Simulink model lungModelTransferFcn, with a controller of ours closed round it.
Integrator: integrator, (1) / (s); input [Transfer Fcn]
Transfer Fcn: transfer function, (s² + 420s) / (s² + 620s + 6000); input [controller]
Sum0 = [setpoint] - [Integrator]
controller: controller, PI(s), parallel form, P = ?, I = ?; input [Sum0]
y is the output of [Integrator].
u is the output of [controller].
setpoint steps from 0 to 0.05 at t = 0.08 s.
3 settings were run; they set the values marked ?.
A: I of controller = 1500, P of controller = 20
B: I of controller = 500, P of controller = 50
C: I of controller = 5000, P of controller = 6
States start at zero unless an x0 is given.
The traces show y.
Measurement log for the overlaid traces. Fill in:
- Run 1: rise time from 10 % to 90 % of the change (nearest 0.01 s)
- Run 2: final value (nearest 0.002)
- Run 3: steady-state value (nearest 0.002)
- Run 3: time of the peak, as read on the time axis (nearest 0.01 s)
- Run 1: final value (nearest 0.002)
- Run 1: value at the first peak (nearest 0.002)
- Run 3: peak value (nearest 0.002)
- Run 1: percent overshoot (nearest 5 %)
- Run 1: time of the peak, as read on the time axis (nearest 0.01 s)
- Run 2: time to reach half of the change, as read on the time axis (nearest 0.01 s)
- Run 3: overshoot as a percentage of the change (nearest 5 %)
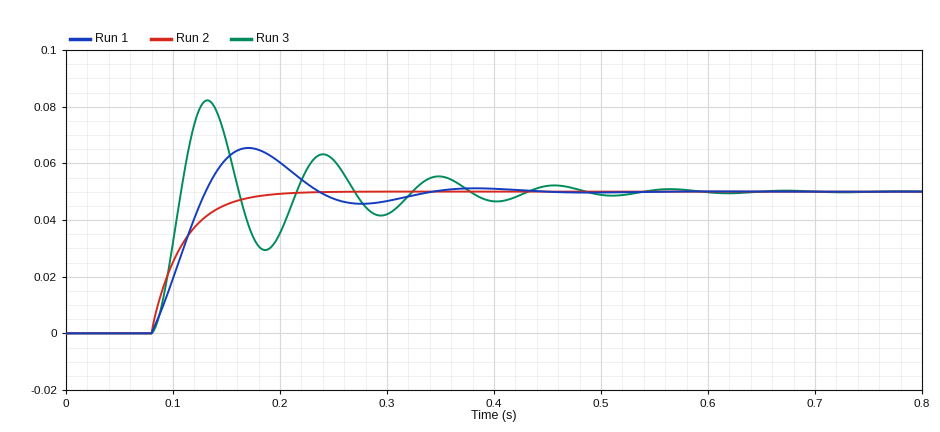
0.04 s
0.050
0.050
0.13 s
0.050
0.066
0.082
30 %
0.17 s
0.10 s
65 %
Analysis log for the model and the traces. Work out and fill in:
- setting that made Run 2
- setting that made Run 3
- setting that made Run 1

B
C
A
